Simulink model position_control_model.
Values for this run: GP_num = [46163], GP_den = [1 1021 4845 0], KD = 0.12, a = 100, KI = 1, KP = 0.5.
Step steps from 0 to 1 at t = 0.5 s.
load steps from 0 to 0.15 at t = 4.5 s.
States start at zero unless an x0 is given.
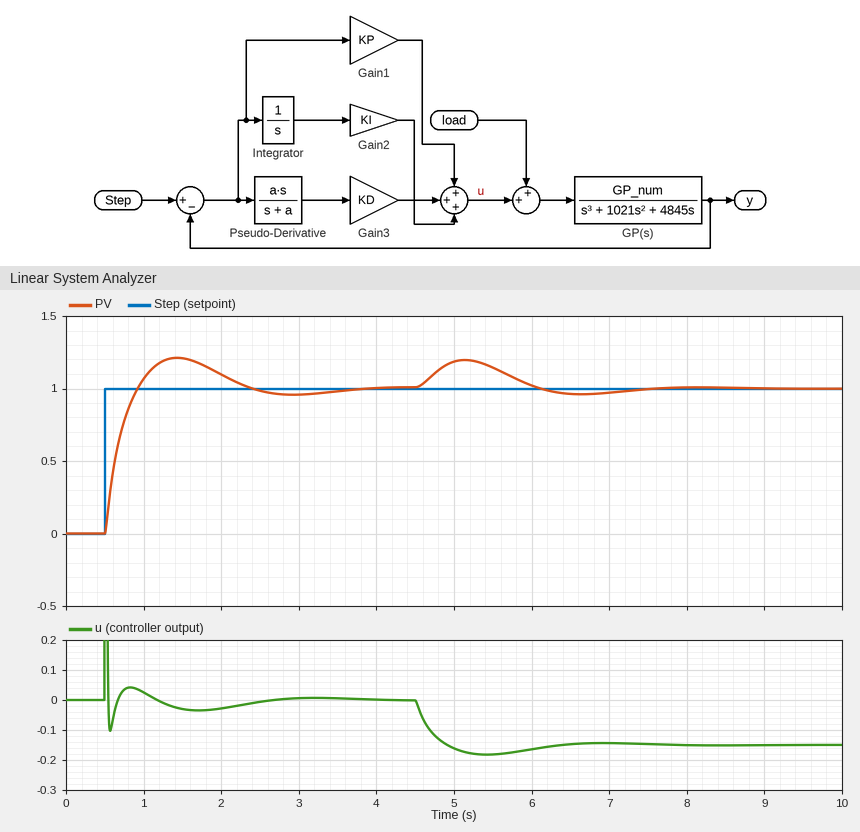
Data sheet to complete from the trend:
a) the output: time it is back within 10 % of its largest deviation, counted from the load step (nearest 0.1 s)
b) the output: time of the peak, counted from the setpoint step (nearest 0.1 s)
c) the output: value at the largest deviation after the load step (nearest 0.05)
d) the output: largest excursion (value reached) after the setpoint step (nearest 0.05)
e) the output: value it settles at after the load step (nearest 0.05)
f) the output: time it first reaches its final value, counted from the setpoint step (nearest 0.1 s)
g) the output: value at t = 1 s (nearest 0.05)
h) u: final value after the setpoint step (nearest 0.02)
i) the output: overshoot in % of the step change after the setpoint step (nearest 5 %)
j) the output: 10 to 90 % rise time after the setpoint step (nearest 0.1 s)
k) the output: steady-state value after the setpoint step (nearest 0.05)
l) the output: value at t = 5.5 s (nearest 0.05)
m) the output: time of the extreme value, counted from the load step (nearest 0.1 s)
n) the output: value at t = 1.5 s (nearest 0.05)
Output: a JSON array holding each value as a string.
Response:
["2.7 s", "0.9 s", "1.20", "1.20", "1.00", "0.4 s", "1.05", "0.00", "20 %", "0.3 s", "1.00", "1.15", "0.6 s", "1.20"]
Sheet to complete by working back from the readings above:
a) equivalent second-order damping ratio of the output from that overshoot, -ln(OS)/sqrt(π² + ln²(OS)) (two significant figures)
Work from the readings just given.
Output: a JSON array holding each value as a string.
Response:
["0.46"]
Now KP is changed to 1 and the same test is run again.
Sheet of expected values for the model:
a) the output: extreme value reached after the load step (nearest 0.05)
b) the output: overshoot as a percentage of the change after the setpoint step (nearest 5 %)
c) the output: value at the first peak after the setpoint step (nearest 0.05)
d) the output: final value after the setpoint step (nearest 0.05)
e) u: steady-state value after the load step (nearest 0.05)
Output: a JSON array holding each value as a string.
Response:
["1.15", "15 %", "1.15", "1.00", "-0.15"]
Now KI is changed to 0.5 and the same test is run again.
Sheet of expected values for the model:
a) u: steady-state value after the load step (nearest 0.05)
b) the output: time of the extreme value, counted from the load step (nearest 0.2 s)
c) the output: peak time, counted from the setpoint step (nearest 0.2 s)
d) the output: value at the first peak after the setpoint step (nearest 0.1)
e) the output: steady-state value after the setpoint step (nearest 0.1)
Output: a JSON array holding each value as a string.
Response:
["-0.15", "0.8 s", "1.2 s", "1.1", "1.0"]
